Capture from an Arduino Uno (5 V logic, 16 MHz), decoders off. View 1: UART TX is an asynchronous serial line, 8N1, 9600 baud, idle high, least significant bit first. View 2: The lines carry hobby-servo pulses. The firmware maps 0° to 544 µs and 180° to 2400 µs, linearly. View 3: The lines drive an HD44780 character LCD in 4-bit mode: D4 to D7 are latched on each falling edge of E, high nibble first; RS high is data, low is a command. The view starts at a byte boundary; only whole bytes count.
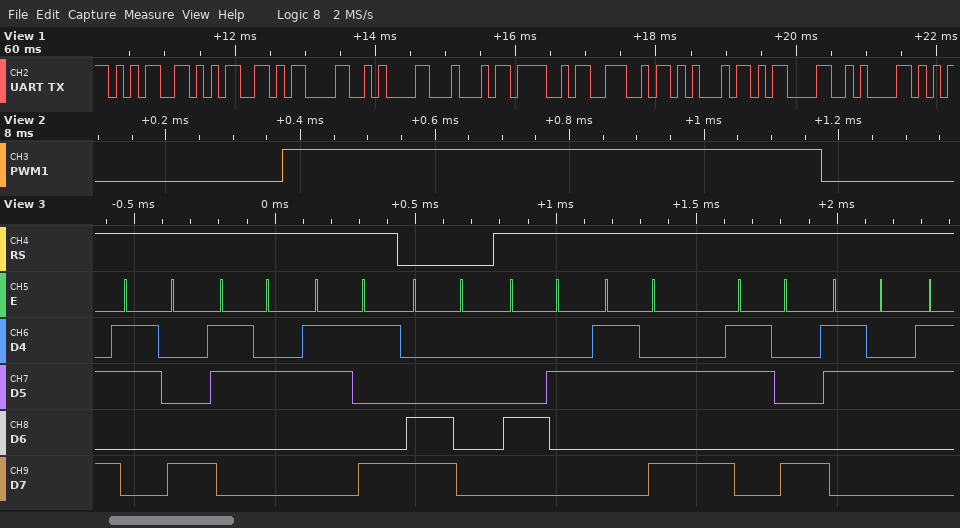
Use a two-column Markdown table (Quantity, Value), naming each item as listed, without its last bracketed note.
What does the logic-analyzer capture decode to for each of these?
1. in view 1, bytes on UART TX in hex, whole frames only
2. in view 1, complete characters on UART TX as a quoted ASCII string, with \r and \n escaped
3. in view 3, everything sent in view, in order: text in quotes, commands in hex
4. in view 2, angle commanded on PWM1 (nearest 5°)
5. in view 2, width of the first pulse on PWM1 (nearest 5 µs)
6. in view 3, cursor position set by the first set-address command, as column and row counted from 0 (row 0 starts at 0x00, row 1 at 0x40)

| Quantity | Value |
|---|---|
| in view 1, bytes on UART TX in hex, whole frames only | 35 35 0D 0A 44 4F 4E 45 0D 0A |
| in view 1, complete characters on UART TX as a quoted ASCII string, with \r and \n escaped | "55\r\nDONE\r\n" |
| in view 3, everything sent in view, in order: text in quotes, commands in hex | "829" 0xC0 "B:82" |
| in view 2, angle commanded on PWM1 | 25° |
| in view 2, width of the first pulse on PWM1 | 800 µs |
| in view 3, cursor position set by the first set-address command, as column and row counted from 0 | column 0, row 1 |
